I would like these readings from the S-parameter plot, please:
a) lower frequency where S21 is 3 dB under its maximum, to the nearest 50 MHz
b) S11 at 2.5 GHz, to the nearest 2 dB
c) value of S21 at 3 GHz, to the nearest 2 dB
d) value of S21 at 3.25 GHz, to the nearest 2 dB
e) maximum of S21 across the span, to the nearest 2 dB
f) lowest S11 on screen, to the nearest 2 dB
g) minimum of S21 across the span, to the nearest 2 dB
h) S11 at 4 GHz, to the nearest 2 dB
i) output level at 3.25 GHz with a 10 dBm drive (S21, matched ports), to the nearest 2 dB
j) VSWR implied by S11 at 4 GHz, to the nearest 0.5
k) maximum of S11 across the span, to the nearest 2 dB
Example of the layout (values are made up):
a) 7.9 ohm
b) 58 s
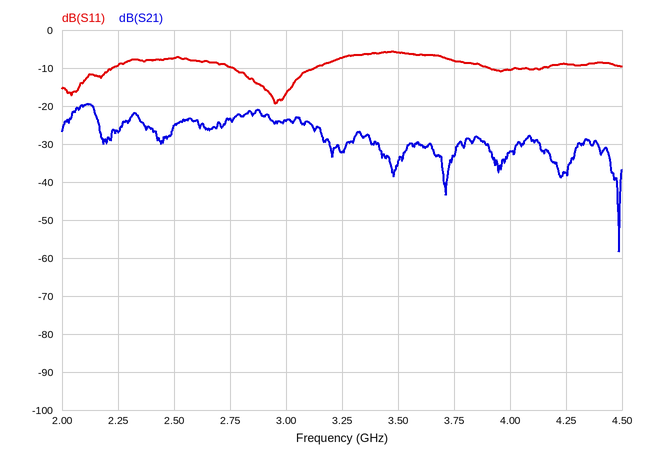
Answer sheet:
a) 2.05 GHz
b) -8 dB
c) -24 dB
d) -32 dB
e) -20 dB
f) -20 dB
g) -58 dB
h) -10 dB
i) -22 dBm
j) 2.0
k) -6 dB
